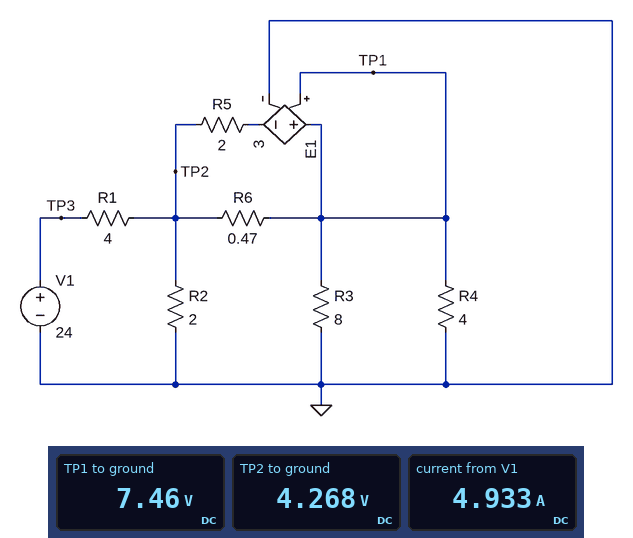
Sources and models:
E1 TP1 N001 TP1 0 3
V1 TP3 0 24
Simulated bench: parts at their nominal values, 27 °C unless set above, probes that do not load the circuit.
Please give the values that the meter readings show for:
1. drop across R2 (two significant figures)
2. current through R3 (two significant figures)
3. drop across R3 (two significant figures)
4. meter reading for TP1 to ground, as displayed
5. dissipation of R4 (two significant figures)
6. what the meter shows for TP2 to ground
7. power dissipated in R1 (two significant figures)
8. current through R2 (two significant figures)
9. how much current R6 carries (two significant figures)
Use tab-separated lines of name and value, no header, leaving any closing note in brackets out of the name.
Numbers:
drop across R2	4.3 V
current through R3	930 mA
drop across R3	7.5 V
meter reading for TP1 to ground, as displayed	7.46 V
dissipation of R4	14 W
what the meter shows for TP2 to ground	4.268 V
power dissipated in R1	97 W
current through R2	2.1 A
how much current R6 carries	6.8 A
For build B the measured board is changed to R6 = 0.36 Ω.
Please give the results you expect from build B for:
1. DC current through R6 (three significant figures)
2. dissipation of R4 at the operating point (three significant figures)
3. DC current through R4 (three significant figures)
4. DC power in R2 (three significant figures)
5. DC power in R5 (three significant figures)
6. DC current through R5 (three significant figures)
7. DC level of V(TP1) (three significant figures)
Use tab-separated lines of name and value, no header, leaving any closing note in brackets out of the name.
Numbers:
DC current through R6	6.59 A
dissipation of R4 at the operating point	12.0 W
DC current through R4	1.73 A
DC power in R2	10.3 W
DC power in R5	169 W
DC current through R5	9.19 A
DC level of V(TP1)	6.92 V
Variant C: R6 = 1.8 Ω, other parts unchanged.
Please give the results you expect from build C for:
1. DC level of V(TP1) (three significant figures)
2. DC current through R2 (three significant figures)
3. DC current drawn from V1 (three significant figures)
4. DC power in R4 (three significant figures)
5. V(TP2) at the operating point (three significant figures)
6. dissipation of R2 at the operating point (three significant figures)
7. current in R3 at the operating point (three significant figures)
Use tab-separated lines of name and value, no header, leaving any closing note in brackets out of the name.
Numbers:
DC level of V(TP1)	18.4 V
DC current through R2	606 mA
DC current drawn from V1	6.30 A
DC power in R4	84.9 W
V(TP2) at the operating point	-1.21 V
dissipation of R2 at the operating point	735 mW
current in R3 at the operating point	2.30 A
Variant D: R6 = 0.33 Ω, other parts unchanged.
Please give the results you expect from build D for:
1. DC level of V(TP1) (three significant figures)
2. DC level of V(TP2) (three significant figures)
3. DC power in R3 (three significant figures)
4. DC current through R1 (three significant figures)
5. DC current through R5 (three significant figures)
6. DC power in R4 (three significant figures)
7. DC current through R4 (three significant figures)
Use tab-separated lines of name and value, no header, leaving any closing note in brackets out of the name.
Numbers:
DC level of V(TP1)	6.77 V
DC level of V(TP2)	4.61 V
DC power in R3	5.73 W
DC current through R1	4.85 A
DC current through R5	9.08 A
DC power in R4	11.5 W
DC current through R4	1.69 A
